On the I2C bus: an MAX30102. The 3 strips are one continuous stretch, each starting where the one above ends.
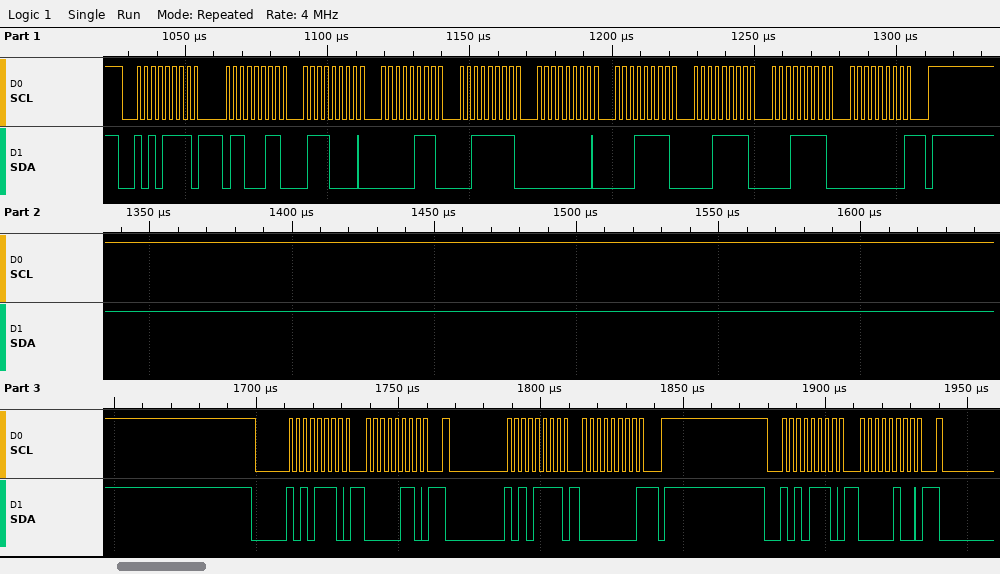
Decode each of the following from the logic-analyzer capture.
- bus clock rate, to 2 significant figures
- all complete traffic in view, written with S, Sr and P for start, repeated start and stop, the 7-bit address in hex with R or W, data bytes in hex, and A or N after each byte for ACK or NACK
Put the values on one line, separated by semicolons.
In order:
400 kHz; S 57R A 63 A 70 A 07 A 3F A 00 A 1F A 1F A 1F A 00 N P S 57W A 06 A Sr 57R A 00 N P S 57W A 04 A
